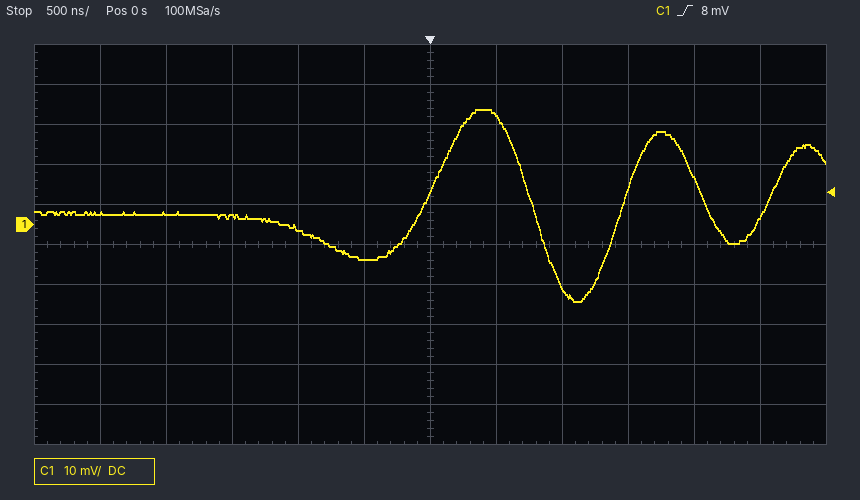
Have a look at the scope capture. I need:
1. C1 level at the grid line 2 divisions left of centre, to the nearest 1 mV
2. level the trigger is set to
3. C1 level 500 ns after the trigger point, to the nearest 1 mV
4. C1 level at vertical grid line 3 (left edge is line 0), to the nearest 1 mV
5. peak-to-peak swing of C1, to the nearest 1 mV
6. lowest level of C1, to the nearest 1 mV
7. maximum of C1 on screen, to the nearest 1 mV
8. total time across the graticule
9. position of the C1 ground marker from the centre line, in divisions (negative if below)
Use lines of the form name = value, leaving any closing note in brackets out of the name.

C1 level at the grid line 2 divisions left of centre, to the nearest 1 mV = -1 mV
level the trigger is set to = 8 mV
C1 level 500 ns after the trigger point, to the nearest 1 mV = 27 mV
C1 level at vertical grid line 3 (left edge is line 0), to the nearest 1 mV = 2 mV
peak-to-peak swing of C1, to the nearest 1 mV = 48 mV
lowest level of C1, to the nearest 1 mV = -19 mV
maximum of C1 on screen, to the nearest 1 mV = 29 mV
total time across the graticule = 6 µs
position of the C1 ground marker from the centre line, in divisions = +0.5 div
